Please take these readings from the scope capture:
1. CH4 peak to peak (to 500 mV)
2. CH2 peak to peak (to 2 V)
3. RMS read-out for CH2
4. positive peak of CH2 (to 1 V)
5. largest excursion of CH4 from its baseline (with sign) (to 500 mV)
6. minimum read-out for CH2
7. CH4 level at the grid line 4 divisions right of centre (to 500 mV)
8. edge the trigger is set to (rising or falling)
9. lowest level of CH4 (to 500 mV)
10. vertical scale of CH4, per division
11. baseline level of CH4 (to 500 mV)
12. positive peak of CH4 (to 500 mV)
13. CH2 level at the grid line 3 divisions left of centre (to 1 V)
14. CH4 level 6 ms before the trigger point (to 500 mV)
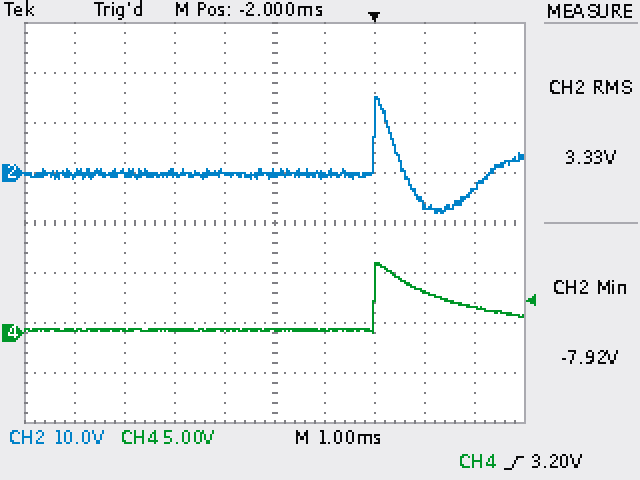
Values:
7.0 V
24 V
3.33 V
15 V
+6.5 V
-7.92 V
2.5 V
rising
0.0 V
5 V
500 mV
7.0 V
0 V
500 mV
